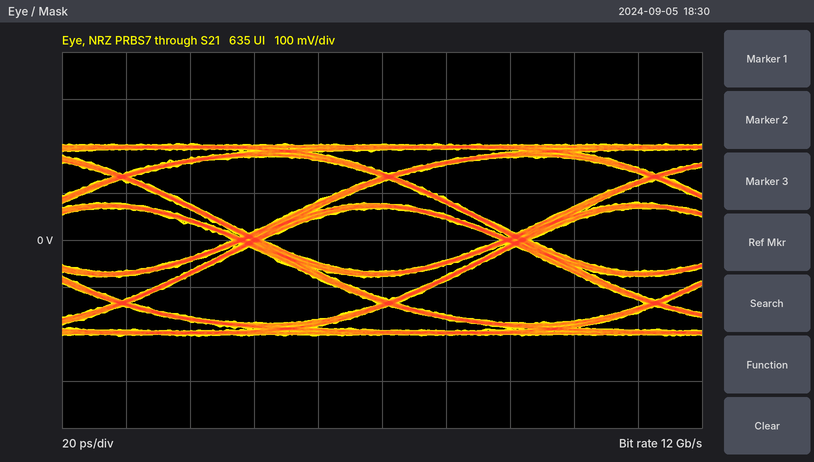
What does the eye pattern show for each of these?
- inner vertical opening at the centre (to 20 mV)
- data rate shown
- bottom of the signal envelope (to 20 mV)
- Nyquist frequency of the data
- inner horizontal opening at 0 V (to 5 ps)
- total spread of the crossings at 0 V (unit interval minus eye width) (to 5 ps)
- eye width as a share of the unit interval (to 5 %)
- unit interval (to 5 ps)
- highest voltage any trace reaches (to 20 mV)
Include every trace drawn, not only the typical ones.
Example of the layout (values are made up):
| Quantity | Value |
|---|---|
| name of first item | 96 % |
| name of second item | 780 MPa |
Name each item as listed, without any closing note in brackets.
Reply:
| Quantity | Value |
|---|---|
| inner vertical opening at the centre | 140 mV |
| data rate shown | 12 Gb/s |
| bottom of the signal envelope | -200 mV |
| Nyquist frequency of the data | 6 GHz |
| inner horizontal opening at 0 V | 75 ps |
| total spread of the crossings at 0 V (unit interval minus eye width) | 10 ps |
| eye width as a share of the unit interval | 90 % |
| unit interval | 85 ps |
| highest voltage any trace reaches | 200 mV |
